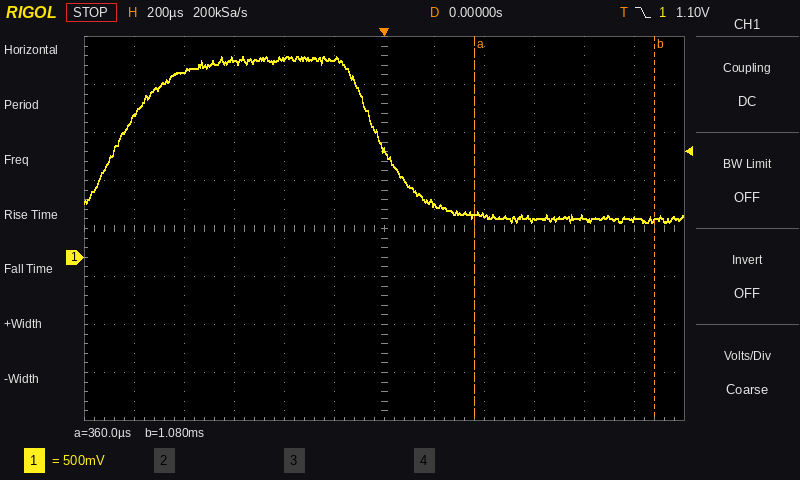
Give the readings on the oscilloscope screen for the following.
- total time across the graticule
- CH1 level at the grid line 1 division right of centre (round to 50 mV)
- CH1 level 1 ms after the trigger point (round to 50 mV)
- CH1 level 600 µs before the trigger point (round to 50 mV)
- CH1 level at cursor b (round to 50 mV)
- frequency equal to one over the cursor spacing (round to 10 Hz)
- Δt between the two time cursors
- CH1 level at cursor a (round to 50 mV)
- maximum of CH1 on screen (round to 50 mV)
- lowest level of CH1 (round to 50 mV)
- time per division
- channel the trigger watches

2.4 ms
550 mV
400 mV
2.05 V
400 mV
1.39 kHz
720 µs
450 mV
2.10 V
350 mV
200 µs
CH1
